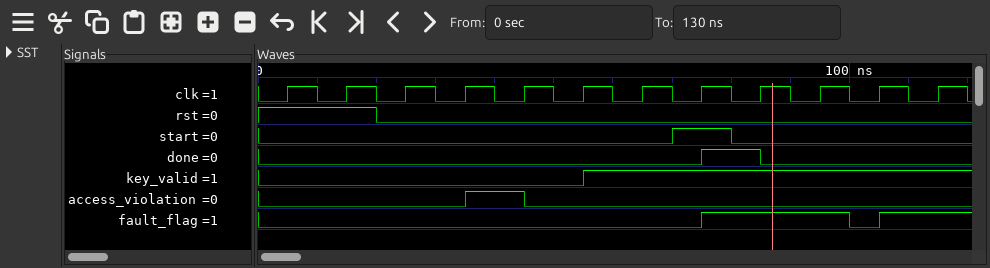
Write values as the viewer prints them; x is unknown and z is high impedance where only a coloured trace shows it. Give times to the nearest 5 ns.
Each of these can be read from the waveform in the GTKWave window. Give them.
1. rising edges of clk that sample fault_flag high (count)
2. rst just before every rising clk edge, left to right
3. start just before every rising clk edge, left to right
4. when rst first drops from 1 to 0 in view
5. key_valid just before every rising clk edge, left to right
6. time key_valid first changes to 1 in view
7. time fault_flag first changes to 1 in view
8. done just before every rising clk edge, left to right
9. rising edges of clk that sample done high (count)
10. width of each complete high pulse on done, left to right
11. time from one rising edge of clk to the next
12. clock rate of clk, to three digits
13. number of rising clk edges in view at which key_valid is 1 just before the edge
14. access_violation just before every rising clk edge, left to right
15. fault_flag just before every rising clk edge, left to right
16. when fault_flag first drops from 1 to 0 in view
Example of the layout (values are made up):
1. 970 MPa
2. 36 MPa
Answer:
1. 3
2. 1 1 0 0 0 0 0 0 0 0 0 0
3. 0 0 0 0 0 0 0 1 0 0 0 0
4. 20 ns
5. 0 0 0 0 0 0 1 1 1 1 1 1
6. 55 ns
7. 75 ns
8. 0 0 0 0 0 0 0 0 1 0 0 0
9. 1
10. 10 ns
11. 10 ns
12. 100 MHz
13. 6
14. 0 0 0 0 1 0 0 0 0 0 0 0
15. 0 0 0 0 0 0 0 0 1 1 0 1
16. 100 ns
